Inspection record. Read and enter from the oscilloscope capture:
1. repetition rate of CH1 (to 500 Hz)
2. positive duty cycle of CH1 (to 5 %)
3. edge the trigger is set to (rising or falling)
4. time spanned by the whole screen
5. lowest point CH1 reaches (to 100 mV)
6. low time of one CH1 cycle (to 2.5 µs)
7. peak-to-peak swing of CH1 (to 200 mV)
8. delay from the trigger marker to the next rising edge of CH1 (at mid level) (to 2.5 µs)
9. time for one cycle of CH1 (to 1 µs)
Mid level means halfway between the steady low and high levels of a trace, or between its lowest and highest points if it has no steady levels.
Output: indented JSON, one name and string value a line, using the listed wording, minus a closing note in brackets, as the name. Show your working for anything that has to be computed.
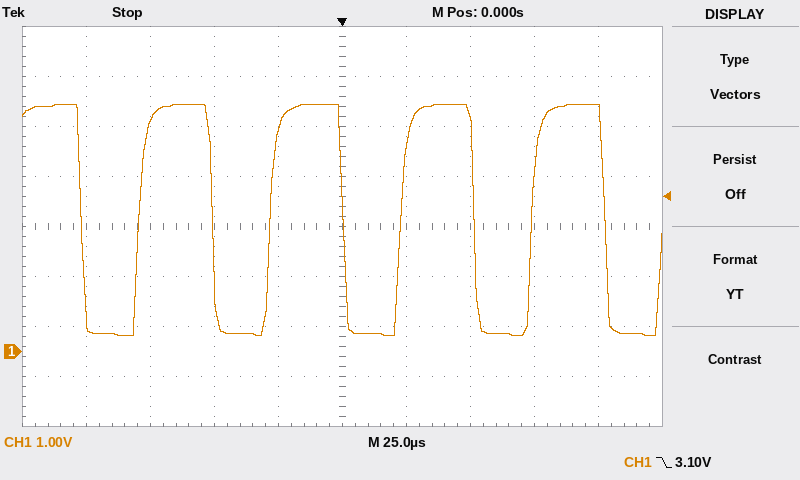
{
  "repetition rate of CH1": "1 / 51 µs ≈ 19.6 kHz, so 19.5 kHz to the nearest 500 Hz",
  "positive duty cycle of CH1": "55 %",
  "edge the trigger is set to": "falling",
  "time spanned by the whole screen": "250 µs",
  "lowest point CH1 reaches": "300 mV",
  "low time of one CH1 cycle": "22.5 µs",
  "peak-to-peak swing of CH1": "4.6 V",
  "delay from the trigger marker to the next rising edge of CH1 (at mid level)": "22.5 µs",
  "time for one cycle of CH1": "51 µs"
}
